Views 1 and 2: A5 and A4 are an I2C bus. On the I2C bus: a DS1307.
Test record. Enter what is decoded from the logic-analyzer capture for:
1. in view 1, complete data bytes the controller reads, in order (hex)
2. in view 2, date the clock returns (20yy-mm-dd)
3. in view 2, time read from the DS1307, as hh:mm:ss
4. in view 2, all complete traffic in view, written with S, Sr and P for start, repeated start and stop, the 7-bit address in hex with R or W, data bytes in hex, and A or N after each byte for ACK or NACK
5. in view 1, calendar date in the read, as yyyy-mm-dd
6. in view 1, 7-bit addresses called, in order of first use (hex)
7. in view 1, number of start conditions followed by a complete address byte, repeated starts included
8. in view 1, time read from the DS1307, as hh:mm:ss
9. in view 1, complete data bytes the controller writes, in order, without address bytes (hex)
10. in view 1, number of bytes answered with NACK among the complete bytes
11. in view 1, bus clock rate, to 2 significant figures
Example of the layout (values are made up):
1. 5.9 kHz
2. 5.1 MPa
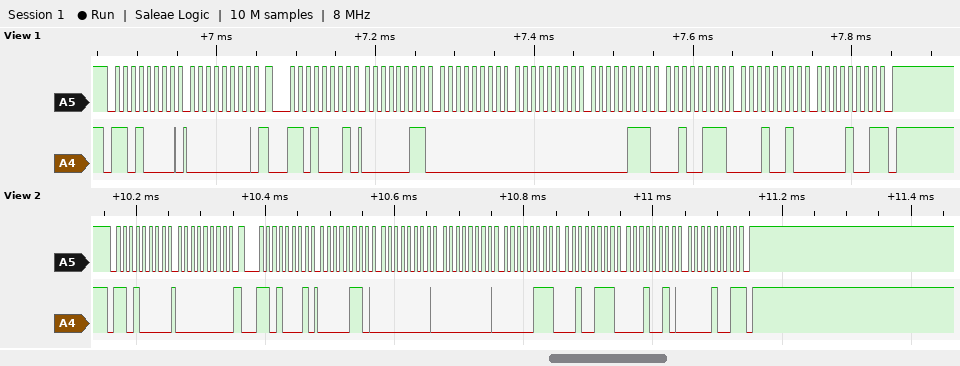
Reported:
1. 03 00 00 07 27 12 09
2. 2009-12-27
3. 00:00:06
4. S 68W A 00 A Sr 68R A 06 A 00 A 00 A 07 A 27 A 12 A 09 N P
5. 2009-12-27
6. 0x68
7. 2
8. 00:00:03
9. 00
10. 1
11. 100 kHz
